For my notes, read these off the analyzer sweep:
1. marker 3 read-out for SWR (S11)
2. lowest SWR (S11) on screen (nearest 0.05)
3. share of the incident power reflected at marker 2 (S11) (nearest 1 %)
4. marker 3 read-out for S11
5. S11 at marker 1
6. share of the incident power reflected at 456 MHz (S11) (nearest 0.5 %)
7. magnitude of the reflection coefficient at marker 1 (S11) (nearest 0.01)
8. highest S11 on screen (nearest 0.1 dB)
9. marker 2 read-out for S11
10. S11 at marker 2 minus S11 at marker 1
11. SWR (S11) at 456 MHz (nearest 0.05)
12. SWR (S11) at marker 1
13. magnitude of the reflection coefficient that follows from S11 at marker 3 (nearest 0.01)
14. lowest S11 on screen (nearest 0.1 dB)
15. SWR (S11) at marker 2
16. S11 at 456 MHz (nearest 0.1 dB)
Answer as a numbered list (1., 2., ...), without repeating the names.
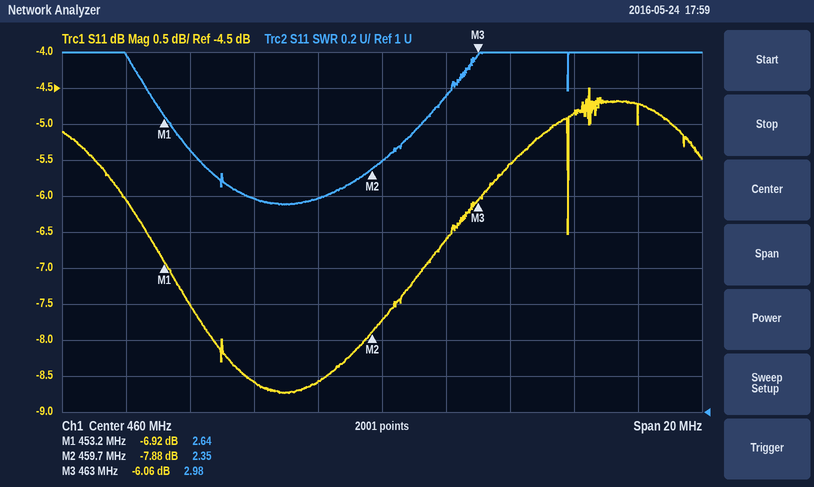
1. 2.98
2. 2.15
3. 16 %
4. -6.06 dB
5. -6.92 dB
6. 14.0 %
7. 0.45
8. -4.5 dB
9. -7.88 dB
10. -0.96 dB
11. 2.20
12. 2.64
13. 0.50
14. -8.7 dB
15. 2.35
16. -8.6 dB
